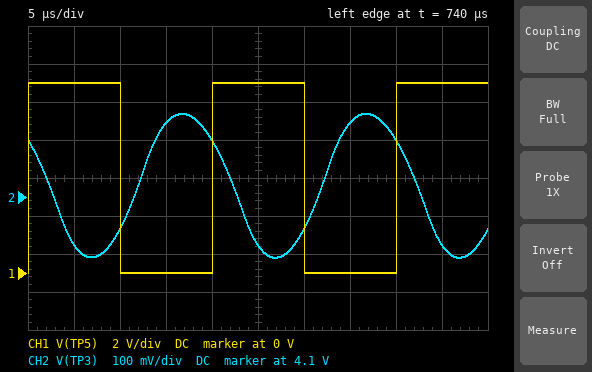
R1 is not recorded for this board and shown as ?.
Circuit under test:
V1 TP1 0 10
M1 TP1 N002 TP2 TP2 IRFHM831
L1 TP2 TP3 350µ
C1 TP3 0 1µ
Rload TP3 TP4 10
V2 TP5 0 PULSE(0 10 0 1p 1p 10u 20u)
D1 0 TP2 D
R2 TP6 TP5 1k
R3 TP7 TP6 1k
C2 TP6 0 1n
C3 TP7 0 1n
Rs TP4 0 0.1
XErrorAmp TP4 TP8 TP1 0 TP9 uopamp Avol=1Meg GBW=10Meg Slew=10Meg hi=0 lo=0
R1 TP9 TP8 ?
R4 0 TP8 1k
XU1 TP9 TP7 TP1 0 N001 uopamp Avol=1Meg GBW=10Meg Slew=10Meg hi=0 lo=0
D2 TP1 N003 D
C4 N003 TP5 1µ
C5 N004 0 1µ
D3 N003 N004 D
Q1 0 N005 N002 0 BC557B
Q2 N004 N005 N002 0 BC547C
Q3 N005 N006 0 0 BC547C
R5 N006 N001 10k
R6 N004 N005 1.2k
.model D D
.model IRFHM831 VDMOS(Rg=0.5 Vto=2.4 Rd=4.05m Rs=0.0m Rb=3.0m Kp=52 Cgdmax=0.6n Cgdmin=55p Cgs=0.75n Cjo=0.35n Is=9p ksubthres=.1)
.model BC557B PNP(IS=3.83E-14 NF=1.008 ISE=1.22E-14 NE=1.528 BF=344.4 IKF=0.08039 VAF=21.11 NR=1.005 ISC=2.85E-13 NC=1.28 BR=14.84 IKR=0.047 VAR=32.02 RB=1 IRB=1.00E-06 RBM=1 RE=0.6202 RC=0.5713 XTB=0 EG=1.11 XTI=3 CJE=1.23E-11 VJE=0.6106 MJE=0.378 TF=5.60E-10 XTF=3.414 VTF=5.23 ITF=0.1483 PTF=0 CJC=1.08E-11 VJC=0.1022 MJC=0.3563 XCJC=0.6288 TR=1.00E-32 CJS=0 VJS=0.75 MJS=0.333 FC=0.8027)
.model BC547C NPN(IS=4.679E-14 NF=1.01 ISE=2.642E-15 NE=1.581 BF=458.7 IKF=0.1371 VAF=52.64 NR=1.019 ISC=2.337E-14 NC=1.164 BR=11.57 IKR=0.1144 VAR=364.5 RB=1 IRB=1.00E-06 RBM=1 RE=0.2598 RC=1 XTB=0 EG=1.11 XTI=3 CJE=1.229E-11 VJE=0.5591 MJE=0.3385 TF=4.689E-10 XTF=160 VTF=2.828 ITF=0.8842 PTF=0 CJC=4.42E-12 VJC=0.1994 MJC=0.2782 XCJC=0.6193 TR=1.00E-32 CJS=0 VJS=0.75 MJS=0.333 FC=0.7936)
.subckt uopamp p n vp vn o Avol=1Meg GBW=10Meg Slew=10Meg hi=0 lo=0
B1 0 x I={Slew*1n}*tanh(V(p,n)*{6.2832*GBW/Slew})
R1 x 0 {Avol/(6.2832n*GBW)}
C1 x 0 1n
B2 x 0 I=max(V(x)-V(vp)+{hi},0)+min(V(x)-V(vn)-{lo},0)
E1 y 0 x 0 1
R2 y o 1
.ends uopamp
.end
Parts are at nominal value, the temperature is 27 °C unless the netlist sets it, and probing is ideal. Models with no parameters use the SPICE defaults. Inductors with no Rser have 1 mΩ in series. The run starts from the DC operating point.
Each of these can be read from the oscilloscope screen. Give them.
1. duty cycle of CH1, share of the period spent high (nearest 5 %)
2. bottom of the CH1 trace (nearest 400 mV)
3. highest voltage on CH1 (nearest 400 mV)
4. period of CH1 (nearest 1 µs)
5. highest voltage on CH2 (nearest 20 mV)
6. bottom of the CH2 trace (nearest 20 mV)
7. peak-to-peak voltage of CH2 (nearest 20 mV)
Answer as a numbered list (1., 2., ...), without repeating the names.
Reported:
1. 50 %
2. 0 V
3. 10.0 V
4. 20 µs
5. 4.32 V
6. 3.94 V
7. 380 mV
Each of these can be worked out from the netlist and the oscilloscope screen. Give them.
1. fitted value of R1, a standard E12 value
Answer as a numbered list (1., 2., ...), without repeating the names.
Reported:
1. 120 kΩ
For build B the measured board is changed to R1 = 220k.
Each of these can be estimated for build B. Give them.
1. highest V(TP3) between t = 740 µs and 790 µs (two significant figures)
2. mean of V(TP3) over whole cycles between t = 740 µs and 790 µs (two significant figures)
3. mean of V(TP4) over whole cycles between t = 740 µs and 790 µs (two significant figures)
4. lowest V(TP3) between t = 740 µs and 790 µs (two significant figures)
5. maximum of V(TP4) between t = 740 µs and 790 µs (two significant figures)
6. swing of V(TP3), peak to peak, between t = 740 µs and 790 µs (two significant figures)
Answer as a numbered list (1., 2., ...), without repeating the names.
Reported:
1. 3.2 V
2. 3.1 V
3. 30 mV
4. 2.9 V
5. 32 mV
6. 350 mV
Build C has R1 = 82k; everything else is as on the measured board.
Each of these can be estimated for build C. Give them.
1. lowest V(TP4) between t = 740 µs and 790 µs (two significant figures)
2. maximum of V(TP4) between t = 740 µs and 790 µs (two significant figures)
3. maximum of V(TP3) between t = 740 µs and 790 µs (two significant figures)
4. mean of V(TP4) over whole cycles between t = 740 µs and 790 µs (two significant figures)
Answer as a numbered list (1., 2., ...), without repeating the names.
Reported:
1. 45 mV
2. 49 mV
3. 4.9 V
4. 47 mV
